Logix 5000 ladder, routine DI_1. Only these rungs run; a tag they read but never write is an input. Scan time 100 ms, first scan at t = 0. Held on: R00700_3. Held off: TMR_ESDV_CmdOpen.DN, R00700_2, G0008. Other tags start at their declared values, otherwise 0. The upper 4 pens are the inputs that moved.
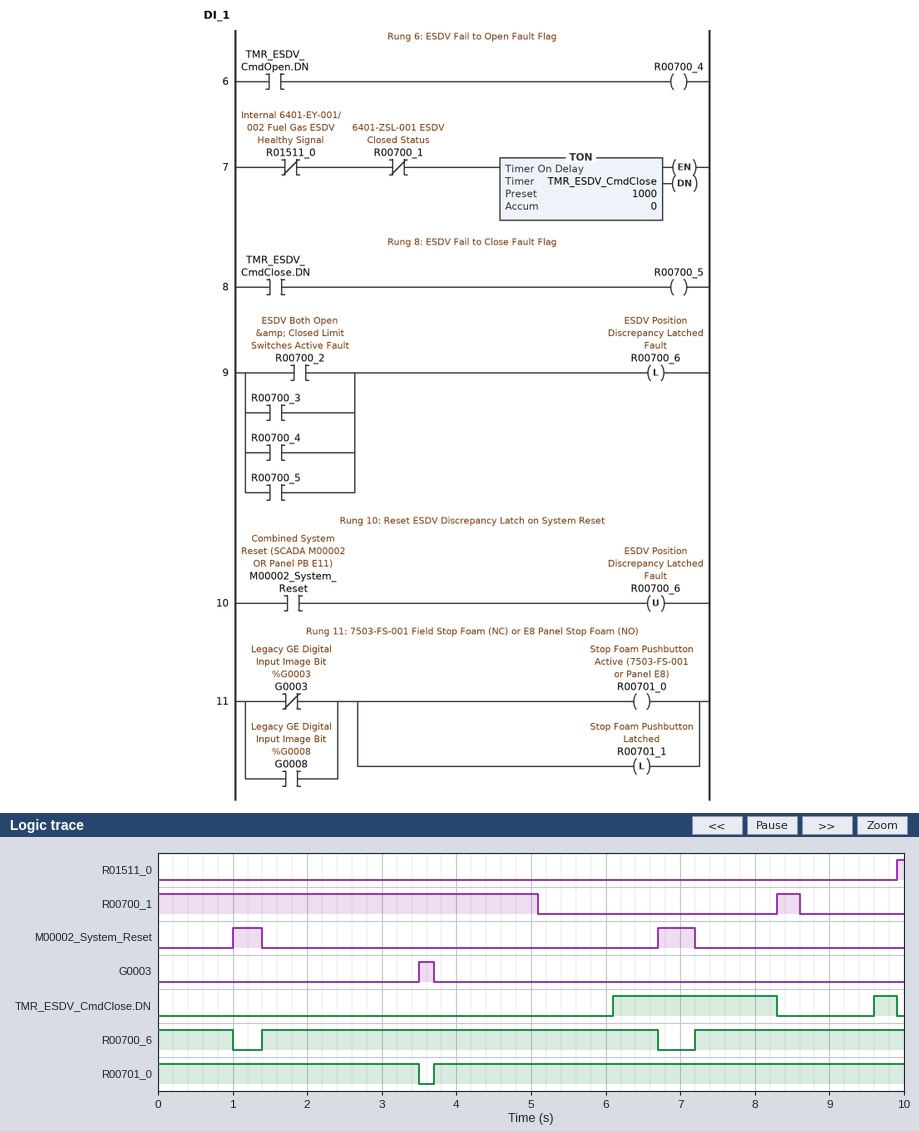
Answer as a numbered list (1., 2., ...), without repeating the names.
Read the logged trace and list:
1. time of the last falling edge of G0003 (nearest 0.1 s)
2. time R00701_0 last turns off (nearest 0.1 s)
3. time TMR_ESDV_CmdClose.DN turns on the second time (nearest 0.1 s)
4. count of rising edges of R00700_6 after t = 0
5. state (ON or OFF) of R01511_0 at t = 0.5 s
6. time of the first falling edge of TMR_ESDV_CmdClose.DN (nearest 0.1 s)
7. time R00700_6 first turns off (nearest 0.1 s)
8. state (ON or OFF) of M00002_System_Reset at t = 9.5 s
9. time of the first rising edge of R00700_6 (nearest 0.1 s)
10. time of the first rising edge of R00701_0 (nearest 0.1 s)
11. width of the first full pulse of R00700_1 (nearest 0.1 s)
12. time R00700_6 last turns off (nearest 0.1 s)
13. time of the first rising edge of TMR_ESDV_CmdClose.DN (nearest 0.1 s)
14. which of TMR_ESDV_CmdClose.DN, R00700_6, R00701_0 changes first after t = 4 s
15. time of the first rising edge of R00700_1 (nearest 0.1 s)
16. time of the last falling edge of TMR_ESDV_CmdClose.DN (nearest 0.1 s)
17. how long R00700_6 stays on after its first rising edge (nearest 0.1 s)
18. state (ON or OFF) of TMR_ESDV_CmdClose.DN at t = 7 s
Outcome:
1. 3.7 s
2. 3.5 s
3. 9.6 s
4. 2
5. OFF
6. 8.3 s
7. 1.0 s
8. OFF
9. 1.4 s
10. 3.7 s
11. 0.3 s
12. 6.7 s
13. 6.1 s
14. TMR_ESDV_CmdClose.DN
15. 8.3 s
16. 9.9 s
17. 5.3 s
18. ON
